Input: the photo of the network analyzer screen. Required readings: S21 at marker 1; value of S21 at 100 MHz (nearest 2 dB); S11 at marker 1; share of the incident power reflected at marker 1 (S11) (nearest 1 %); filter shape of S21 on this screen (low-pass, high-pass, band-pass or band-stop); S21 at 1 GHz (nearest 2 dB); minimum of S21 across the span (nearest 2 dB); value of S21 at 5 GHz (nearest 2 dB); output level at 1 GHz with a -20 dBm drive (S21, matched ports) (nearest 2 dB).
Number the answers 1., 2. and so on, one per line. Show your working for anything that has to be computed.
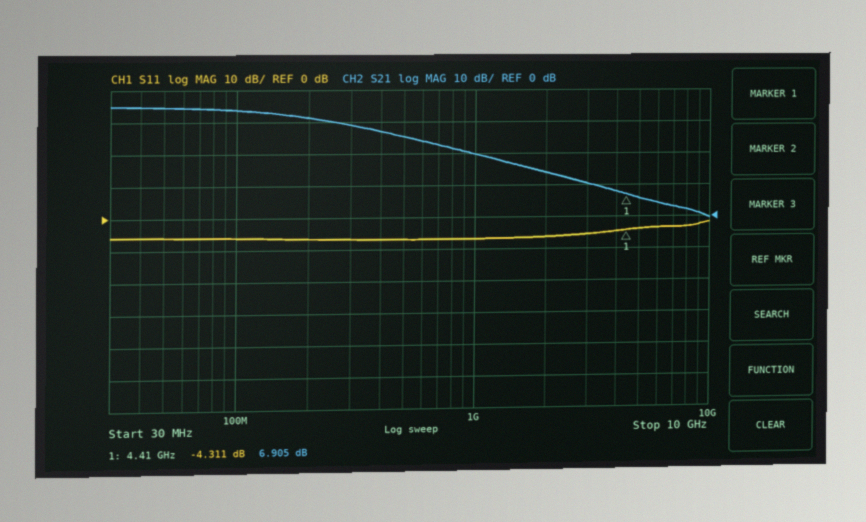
1. 6.905 dB
2. 34 dB
3. -4.311 dB
4. 10^(-4.311/10) ≈ 37 %
5. low-pass
6. 20 dB
7. 0 dB
8. 6 dB
9. -20 dBm + (20 dB) = 0 dBm
